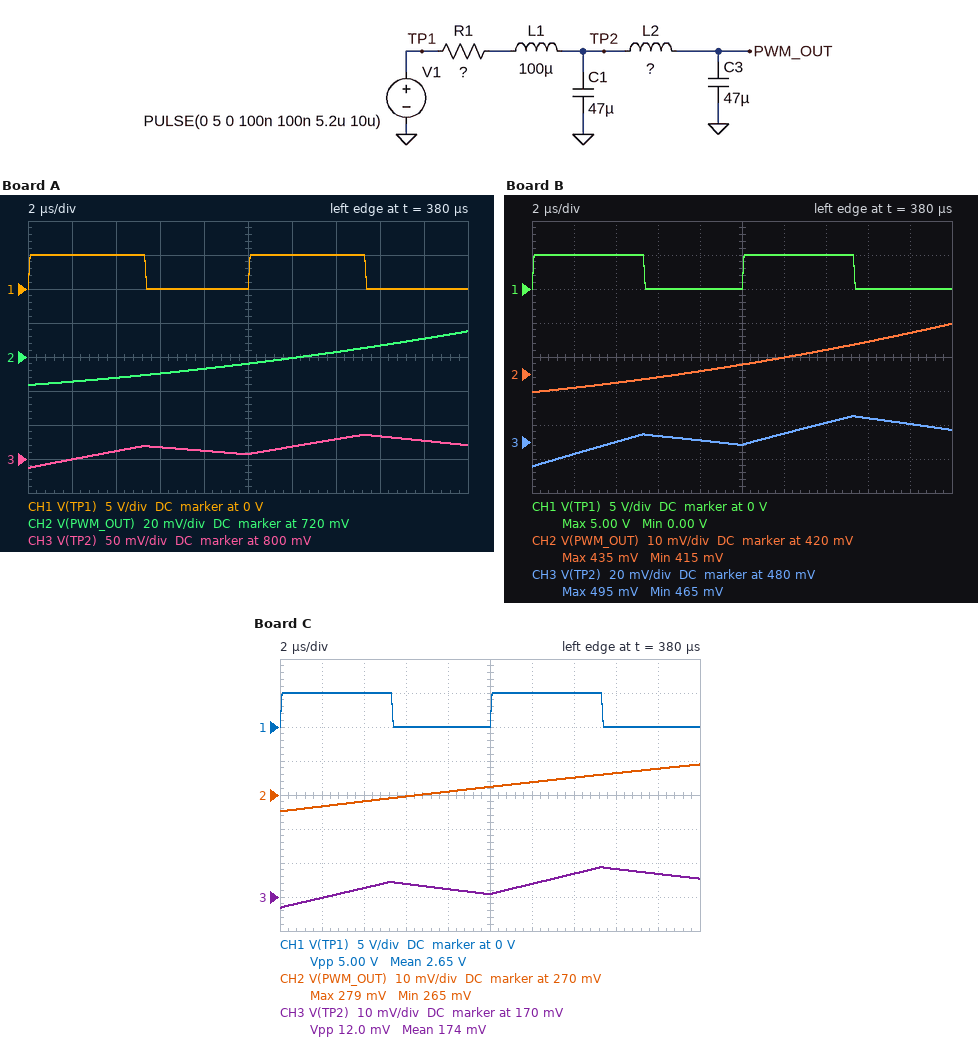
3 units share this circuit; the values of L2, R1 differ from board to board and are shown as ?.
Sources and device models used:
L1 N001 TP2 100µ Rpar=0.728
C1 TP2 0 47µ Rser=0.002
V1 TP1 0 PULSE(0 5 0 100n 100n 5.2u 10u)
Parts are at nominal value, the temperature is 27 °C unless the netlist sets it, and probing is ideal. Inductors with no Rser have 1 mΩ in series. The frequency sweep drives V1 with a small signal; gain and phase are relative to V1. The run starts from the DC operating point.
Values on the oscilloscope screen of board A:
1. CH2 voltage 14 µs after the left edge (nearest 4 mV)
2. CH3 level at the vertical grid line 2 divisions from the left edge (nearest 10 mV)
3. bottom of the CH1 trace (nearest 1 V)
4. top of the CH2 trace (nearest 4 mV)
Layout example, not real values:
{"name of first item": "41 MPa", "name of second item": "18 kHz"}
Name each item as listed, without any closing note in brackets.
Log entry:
{"CH2 voltage 14 µs after the left edge": "724 mV", "CH3 level at the vertical grid line 2 divisions from the left edge": "810 mV", "bottom of the CH1 trace": "0 V", "top of the CH2 trace": "736 mV"}
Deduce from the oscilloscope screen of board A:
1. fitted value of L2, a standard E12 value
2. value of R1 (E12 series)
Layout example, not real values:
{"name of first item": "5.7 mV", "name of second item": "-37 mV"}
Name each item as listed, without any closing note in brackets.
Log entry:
{"fitted value of L2, a standard E12 value": "33 µH", "value of R1": "12 Ω"}
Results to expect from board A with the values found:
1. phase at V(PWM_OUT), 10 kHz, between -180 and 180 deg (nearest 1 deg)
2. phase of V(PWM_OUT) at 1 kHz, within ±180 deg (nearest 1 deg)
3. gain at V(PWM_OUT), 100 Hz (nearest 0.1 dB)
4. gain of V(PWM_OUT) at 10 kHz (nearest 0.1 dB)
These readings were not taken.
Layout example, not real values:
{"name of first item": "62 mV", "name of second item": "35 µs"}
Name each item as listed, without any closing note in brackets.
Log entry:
{"phase at V(PWM_OUT), 10 kHz, between -180 and 180 deg": "92 deg", "phase of V(PWM_OUT) at 1 kHz, within ±180 deg": "-84 deg", "gain at V(PWM_OUT), 100 Hz": "-1.7 dB", "gain of V(PWM_OUT) at 10 kHz": "-43.8 dB"}
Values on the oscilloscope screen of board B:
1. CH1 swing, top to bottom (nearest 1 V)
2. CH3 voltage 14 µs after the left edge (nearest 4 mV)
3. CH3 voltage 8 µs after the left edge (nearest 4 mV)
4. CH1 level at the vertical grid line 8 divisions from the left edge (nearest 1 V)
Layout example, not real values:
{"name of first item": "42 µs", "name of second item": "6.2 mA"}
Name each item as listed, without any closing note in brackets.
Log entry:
{"CH1 swing, top to bottom": "5 V", "CH3 voltage 14 µs after the left edge": "492 mV", "CH3 voltage 8 µs after the left edge": "480 mV", "CH1 level at the vertical grid line 8 divisions from the left edge": "0 V"}
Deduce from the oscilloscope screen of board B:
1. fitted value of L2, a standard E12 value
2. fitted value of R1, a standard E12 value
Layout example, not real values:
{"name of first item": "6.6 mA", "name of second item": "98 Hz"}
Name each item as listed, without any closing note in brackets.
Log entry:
{"fitted value of L2, a standard E12 value": "33 µH", "fitted value of R1, a standard E12 value": "22 Ω"}
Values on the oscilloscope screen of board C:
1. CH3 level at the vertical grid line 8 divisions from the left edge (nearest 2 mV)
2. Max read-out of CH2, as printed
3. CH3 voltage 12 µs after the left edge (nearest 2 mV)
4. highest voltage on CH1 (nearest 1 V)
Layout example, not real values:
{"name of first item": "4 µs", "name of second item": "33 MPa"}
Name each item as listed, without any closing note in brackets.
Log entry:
{"CH3 level at the vertical grid line 8 divisions from the left edge": "178 mV", "Max read-out of CH2, as printed": "279 mV", "CH3 voltage 12 µs after the left edge": "174 mV", "highest voltage on CH1": "5 V"}
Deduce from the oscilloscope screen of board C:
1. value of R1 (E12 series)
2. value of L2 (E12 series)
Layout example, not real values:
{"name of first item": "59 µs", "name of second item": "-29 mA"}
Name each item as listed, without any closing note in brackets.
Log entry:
{"value of R1": "47 Ω", "value of L2": "330 µH"}
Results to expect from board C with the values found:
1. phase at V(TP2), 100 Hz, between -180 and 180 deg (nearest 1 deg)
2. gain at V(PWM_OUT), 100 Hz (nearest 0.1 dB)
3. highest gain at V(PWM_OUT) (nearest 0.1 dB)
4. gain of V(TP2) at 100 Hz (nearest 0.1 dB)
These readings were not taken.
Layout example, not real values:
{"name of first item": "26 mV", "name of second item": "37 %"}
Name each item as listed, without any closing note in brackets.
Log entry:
{"phase at V(TP2), 100 Hz, between -180 and 180 deg": "-70 deg", "gain at V(PWM_OUT), 100 Hz": "-9.4 dB", "highest gain at V(PWM_OUT)": "0 dB", "gain of V(TP2) at 100 Hz": "-9.4 dB"}
